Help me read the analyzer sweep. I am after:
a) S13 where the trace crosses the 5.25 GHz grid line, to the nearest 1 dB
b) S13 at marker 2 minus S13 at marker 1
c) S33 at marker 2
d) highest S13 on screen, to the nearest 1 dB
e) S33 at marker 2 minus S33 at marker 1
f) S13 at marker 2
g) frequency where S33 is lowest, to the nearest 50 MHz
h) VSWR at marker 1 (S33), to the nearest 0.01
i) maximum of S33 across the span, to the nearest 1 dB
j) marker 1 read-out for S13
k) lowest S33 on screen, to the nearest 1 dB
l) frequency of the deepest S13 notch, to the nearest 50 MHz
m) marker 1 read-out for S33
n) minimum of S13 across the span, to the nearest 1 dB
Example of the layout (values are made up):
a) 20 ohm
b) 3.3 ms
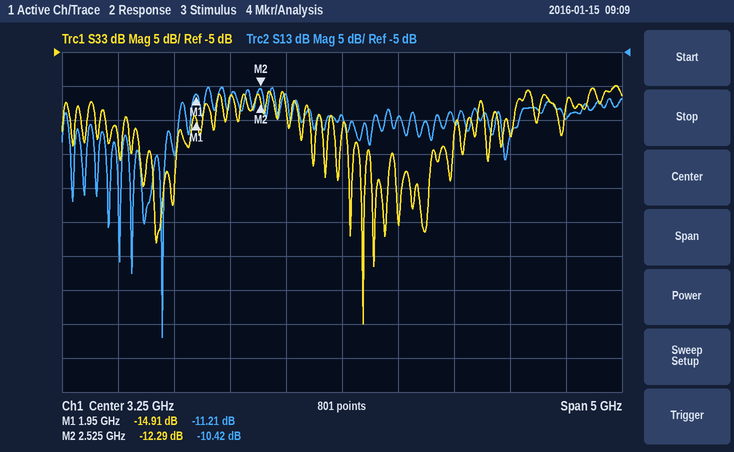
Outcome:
a) -15 dB
b) 0.79 dB
c) -12.29 dB
d) -10 dB
e) 2.62 dB
f) -10.42 dB
g) 3.45 GHz
h) 1.44
i) -10 dB
j) -11.21 dB
k) -45 dB
l) 1.65 GHz
m) -14.91 dB
n) -47 dB
